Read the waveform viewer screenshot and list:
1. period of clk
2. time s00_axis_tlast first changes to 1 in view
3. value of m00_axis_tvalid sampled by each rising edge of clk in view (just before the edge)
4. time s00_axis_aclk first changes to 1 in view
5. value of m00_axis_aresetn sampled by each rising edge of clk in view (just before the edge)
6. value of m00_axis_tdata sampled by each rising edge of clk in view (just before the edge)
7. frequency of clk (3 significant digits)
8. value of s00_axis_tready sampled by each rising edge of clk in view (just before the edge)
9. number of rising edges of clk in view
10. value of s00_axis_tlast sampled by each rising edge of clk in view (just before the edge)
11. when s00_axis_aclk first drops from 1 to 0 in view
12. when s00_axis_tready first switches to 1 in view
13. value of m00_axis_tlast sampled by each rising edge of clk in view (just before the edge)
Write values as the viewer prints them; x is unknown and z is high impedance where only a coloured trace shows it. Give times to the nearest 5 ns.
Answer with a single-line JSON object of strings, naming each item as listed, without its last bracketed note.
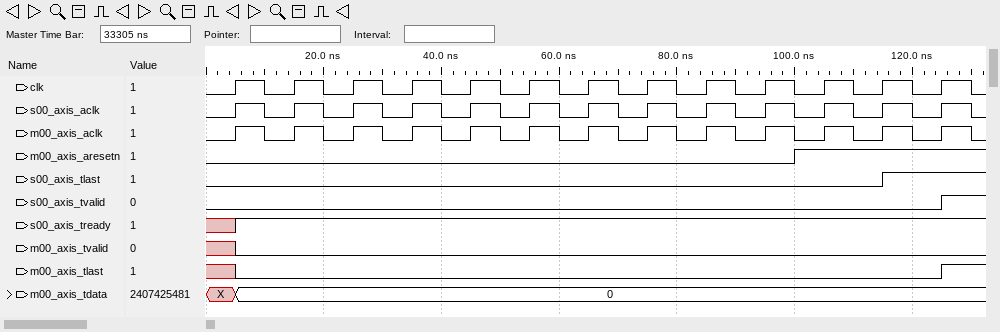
{"period of clk": "10 ns", "time s00_axis_tlast first changes to 1 in view": "115 ns", "value of m00_axis_tvalid sampled by each rising edge of clk in view": "x 0 0 0 0 0 0 0 0 0 0 0 0", "time s00_axis_aclk first changes to 1 in view": "5 ns", "value of m00_axis_aresetn sampled by each rising edge of clk in view": "0 0 0 0 0 0 0 0 0 0 1 1 1", "value of m00_axis_tdata sampled by each rising edge of clk in view": "X, 0, 0, 0, 0, 0, 0, 0, 0, 0, 0, 0, 0", "frequency of clk": "100 MHz", "value of s00_axis_tready sampled by each rising edge of clk in view": "x 1 1 1 1 1 1 1 1 1 1 1 1", "number of rising edges of clk in view": "13", "value of s00_axis_tlast sampled by each rising edge of clk in view": "0 0 0 0 0 0 0 0 0 0 0 0 1", "when s00_axis_aclk first drops from 1 to 0 in view": "10 ns", "when s00_axis_tready first switches to 1 in view": "5 ns", "value of m00_axis_tlast sampled by each rising edge of clk in view": "x 0 0 0 0 0 0 0 0 0 0 0 0"}
